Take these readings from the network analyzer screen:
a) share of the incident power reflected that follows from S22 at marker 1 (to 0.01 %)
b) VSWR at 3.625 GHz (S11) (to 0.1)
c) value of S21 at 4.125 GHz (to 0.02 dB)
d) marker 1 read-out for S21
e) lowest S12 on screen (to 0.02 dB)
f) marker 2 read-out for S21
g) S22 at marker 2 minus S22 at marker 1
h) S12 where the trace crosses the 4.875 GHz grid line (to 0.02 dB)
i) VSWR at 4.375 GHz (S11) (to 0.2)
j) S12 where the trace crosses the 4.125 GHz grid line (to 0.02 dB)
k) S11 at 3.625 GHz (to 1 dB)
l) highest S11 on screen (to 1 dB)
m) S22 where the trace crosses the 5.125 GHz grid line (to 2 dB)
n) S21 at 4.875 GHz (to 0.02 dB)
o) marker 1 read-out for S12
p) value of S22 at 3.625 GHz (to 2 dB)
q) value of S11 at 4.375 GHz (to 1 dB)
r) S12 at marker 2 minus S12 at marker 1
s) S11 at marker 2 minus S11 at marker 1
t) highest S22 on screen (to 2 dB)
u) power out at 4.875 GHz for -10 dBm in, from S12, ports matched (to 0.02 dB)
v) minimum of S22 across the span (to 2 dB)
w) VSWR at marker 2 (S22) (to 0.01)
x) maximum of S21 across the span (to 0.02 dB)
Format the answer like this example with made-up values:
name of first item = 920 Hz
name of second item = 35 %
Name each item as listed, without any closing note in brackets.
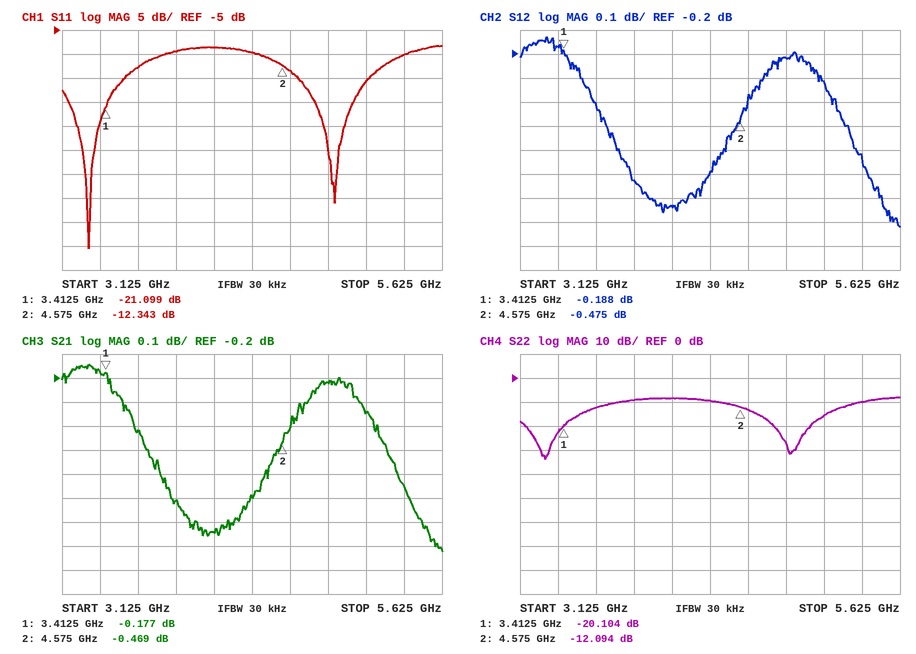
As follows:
share of the incident power reflected that follows from S22 at marker 1 = 0.98 %
VSWR at 3.625 GHz (S11) = 1.6
value of S21 at 4.125 GHz = -0.84 dB
marker 1 read-out for S21 = -0.177 dB
lowest S12 on screen = -0.92 dB
marker 2 read-out for S21 = -0.469 dB
S22 at marker 2 minus S22 at marker 1 = 8.010 dB
S12 where the trace crosses the 4.875 GHz grid line = -0.22 dB
VSWR at 4.375 GHz (S11) = 2.0
S12 where the trace crosses the 4.125 GHz grid line = -0.84 dB
S11 at 3.625 GHz = -13 dB
highest S11 on screen = -8 dB
S22 where the trace crosses the 5.125 GHz grid line = -16 dB
S21 at 4.875 GHz = -0.22 dB
marker 1 read-out for S12 = -0.188 dB
value of S22 at 3.625 GHz = -12 dB
value of S11 at 4.375 GHz = -10 dB
S12 at marker 2 minus S12 at marker 1 = -0.287 dB
S11 at marker 2 minus S11 at marker 1 = 8.756 dB
highest S22 on screen = -8 dB
power out at 4.875 GHz for -10 dBm in, from S12, ports matched = -10.22 dBm
minimum of S22 across the span = -34 dB
VSWR at marker 2 (S22) = 1.66
maximum of S21 across the span = -0.14 dB
